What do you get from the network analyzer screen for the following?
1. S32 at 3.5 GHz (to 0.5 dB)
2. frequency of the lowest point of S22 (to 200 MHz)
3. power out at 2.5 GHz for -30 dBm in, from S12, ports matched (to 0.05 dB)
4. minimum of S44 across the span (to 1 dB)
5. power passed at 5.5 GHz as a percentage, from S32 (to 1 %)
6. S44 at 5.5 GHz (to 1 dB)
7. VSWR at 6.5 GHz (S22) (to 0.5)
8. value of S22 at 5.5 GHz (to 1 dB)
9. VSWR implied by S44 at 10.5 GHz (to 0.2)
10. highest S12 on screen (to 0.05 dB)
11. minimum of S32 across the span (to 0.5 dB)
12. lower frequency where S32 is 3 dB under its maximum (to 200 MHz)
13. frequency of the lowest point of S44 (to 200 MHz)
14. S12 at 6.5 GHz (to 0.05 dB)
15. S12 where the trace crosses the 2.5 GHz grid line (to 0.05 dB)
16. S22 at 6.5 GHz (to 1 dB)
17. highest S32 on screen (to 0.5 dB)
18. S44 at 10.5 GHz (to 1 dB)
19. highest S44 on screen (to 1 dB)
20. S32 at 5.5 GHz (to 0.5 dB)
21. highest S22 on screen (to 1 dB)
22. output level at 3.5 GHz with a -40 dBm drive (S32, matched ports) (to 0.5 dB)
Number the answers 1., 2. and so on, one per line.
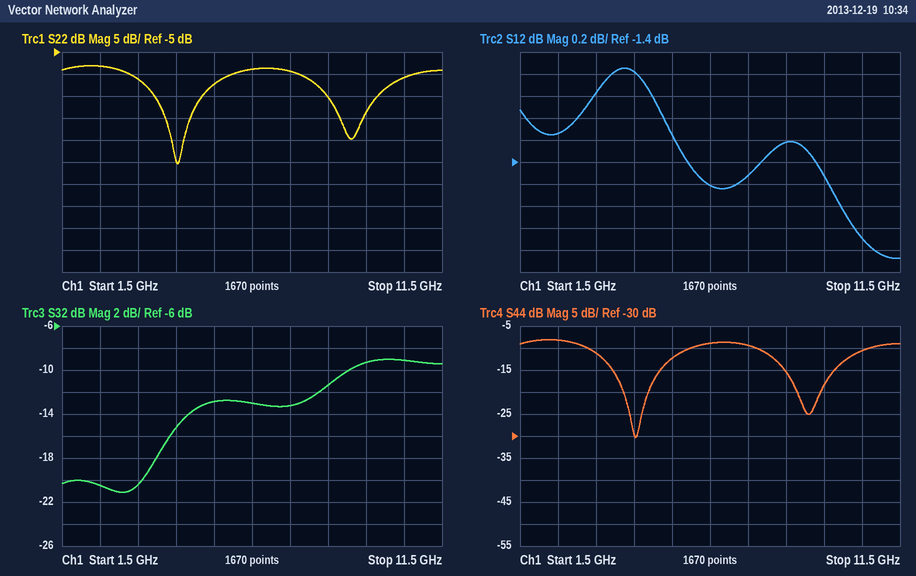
1. -20.5 dB
2. 4.6 GHz
3. -31.15 dBm
4. -30 dB
5. 5 %
6. -12 dB
7. 2.0
8. -12 dB
9. 1.8
10. -0.55 dB
11. -21.0 dB
12. 8.2 GHz
13. 4.6 GHz
14. -1.60 dB
15. -1.15 dB
16. -9 dB
17. -9.0 dB
18. -11 dB
19. -8 dB
20. -13.0 dB
21. -8 dB
22. -60.5 dBm
